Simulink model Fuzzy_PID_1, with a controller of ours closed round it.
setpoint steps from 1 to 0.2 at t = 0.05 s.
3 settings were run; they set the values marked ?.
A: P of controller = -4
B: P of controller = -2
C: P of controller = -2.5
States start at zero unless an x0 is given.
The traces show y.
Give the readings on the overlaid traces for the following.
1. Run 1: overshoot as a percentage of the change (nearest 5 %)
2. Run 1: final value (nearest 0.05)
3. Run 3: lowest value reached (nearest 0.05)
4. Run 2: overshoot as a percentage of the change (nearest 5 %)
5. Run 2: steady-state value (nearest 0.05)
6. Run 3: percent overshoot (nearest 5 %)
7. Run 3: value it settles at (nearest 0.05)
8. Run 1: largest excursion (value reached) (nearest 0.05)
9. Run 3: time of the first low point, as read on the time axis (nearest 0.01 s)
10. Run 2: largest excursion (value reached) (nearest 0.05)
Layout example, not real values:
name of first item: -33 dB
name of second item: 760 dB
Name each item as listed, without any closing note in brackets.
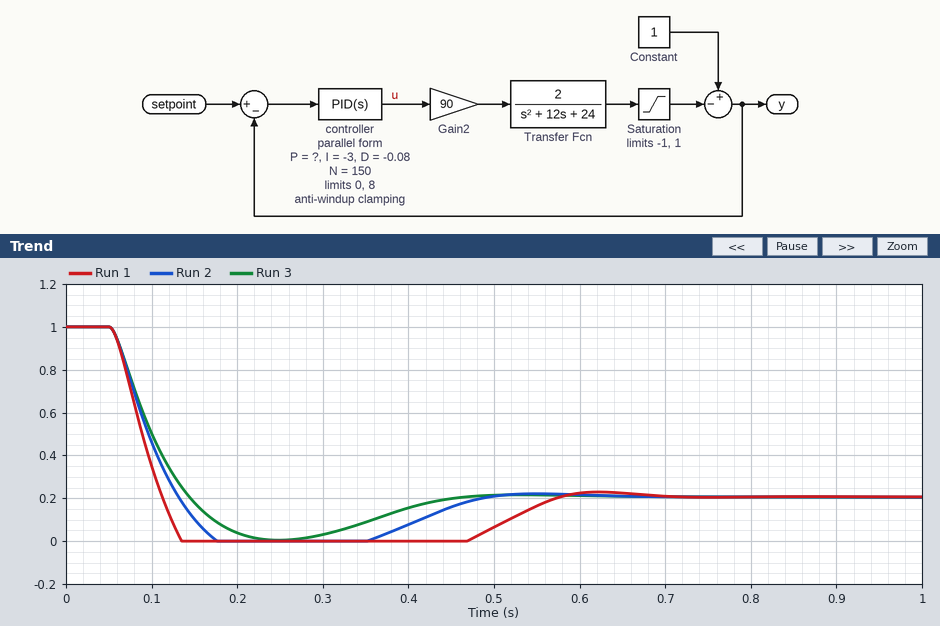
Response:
Run 1: overshoot as a percentage of the change: 25 %
Run 1: final value: 0.20
Run 3: lowest value reached: 0.00
Run 2: overshoot as a percentage of the change: 25 %
Run 2: steady-state value: 0.20
Run 3: percent overshoot: 25 %
Run 3: value it settles at: 0.20
Run 1: largest excursion (value reached): 0.00
Run 3: time of the first low point, as read on the time axis: 0.25 s
Run 2: largest excursion (value reached): 0.00
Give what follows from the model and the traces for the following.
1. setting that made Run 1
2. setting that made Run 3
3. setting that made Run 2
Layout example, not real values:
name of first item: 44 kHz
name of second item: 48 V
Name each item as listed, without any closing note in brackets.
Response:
setting that made Run 1: A
setting that made Run 3: B
setting that made Run 2: C
